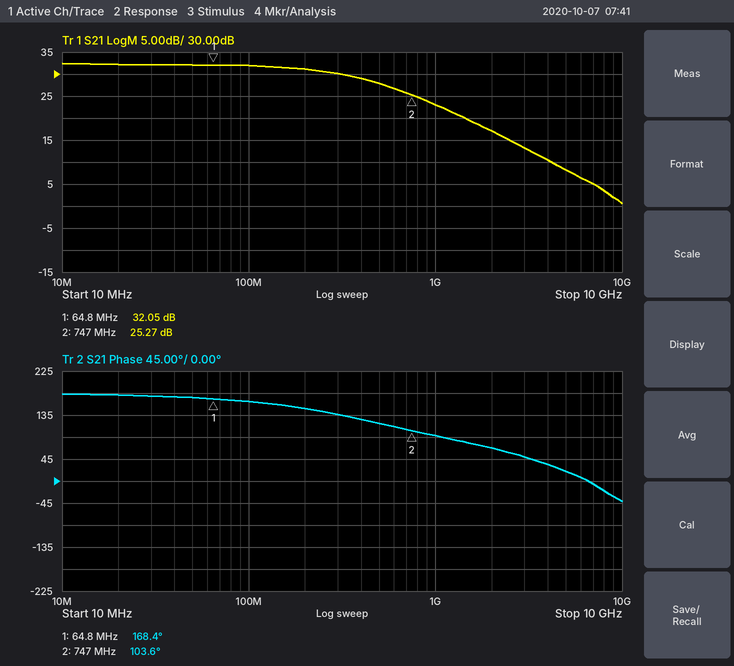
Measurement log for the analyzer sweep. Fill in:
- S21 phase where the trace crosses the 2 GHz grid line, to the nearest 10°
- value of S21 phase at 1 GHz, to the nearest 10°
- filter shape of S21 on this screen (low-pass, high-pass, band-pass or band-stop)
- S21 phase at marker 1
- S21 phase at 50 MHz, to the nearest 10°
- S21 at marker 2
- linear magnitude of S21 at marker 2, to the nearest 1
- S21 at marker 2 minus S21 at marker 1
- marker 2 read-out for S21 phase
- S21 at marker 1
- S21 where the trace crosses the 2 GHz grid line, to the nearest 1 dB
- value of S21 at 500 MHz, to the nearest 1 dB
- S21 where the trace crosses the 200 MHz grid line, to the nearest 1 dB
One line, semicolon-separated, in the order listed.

70°; 90°; low-pass; 168.4°; 170°; 25.27 dB; 18; -6.78 dB; 103.6°; 32.05 dB; 17 dB; 28 dB; 31 dB
